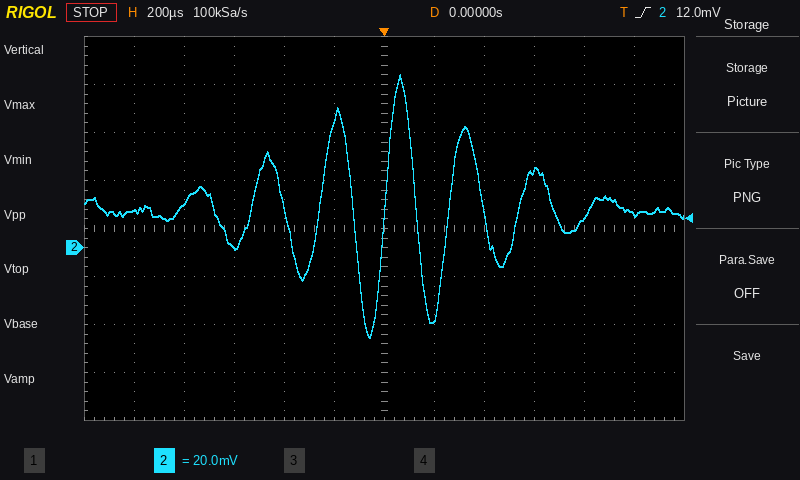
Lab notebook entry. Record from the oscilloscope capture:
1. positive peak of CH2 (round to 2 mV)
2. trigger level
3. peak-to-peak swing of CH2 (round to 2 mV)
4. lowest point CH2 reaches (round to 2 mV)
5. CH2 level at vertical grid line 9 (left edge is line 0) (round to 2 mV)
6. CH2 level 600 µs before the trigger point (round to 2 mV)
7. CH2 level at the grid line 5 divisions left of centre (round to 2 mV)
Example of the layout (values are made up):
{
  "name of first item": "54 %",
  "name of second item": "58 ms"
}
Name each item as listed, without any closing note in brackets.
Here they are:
{
  "positive peak of CH2": "72 mV",
  "trigger level": "12.0 mV",
  "peak-to-peak swing of CH2": "110 mV",
  "lowest point CH2 reaches": "-38 mV",
  "CH2 level at vertical grid line 9 (left edge is line 0)": "32 mV",
  "CH2 level 600 µs before the trigger point": "0 mV",
  "CH2 level at the grid line 5 divisions left of centre": "16 mV"
}
